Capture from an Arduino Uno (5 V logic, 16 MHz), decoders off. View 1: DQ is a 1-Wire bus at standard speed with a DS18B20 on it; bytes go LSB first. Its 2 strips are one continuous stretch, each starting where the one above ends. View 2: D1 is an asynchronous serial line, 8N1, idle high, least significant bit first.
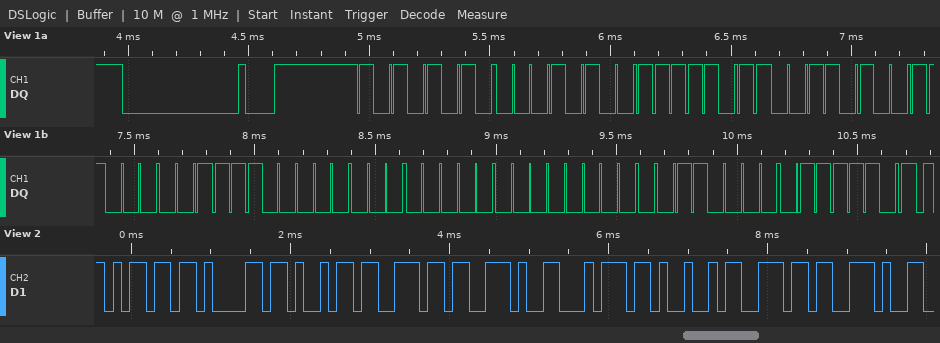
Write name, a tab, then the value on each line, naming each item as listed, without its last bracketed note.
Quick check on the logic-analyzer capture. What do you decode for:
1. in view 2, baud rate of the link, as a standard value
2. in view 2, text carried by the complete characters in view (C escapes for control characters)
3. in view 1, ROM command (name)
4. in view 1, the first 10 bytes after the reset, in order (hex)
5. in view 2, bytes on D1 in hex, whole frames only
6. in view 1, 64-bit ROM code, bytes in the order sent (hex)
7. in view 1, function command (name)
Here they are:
in view 2, baud rate of the link, as a standard value	9600 baud
in view 2, text carried by the complete characters in view	"main.tIn."
in view 1, ROM command	Match ROM
in view 1, the first 10 bytes after the reset, in order	55 28 DF 2C 83 07 00 00 0C BE
in view 2, bytes on D1 in hex, whole frames only	6D 61 69 6E 2E 74 49 6E 2E
in view 1, 64-bit ROM code, bytes in the order sent	28 DF 2C 83 07 00 00 0C
in view 1, function command	Read Scratchpad
